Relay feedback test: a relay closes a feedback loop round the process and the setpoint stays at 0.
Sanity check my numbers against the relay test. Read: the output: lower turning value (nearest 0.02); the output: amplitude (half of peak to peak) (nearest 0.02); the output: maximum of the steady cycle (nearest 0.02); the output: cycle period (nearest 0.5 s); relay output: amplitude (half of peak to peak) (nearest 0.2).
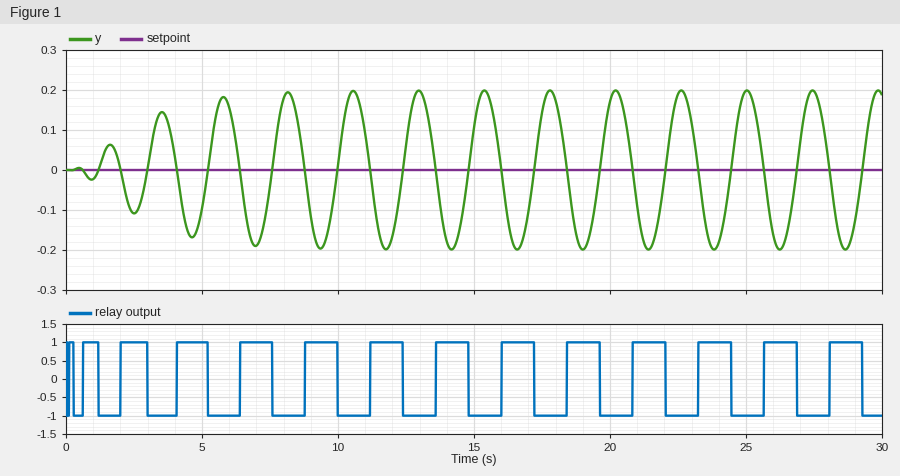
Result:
-0.20
0.20
0.20
2.5 s
1.0
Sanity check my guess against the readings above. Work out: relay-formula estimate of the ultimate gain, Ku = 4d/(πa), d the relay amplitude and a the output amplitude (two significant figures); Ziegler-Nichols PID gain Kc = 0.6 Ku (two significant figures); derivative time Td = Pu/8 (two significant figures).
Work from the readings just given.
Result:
6.4
3.8
0.31 s
